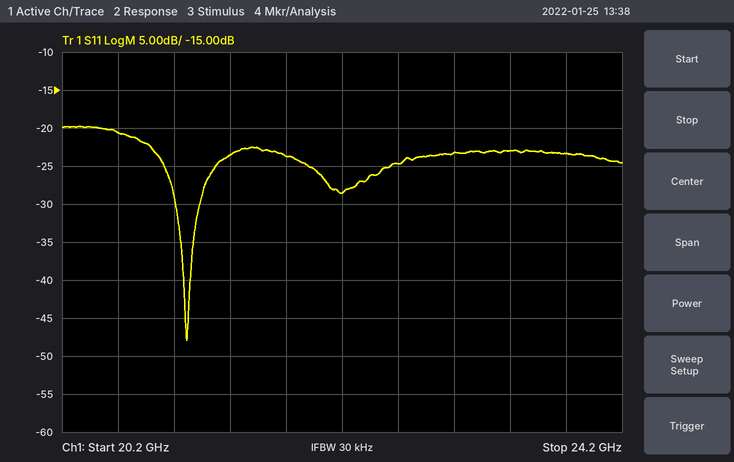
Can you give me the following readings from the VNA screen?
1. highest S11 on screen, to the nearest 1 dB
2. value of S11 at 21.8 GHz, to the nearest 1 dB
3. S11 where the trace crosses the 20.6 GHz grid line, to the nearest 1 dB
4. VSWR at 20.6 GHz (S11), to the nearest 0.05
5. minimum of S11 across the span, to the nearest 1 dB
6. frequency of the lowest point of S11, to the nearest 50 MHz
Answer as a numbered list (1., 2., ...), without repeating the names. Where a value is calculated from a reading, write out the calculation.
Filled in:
1. -20 dB
2. -24 dB
3. -21 dB
4. |Γ| = 10^(-21/20) = 0.0891; VSWR = (1 + 0.0891)/(1 − 0.0891) ≈ 1.20
5. -48 dB
6. 21.10 GHz
